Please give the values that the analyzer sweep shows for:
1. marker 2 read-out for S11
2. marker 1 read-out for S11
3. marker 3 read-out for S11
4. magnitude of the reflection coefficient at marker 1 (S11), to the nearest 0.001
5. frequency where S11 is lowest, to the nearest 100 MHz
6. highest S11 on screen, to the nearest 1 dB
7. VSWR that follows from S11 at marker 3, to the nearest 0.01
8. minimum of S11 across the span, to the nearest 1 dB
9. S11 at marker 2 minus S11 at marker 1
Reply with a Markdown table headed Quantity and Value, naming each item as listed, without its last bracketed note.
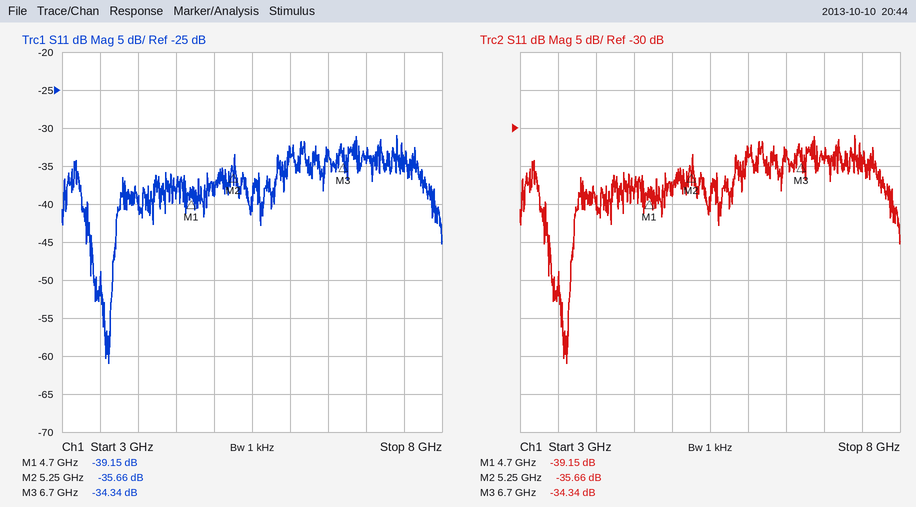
| Quantity | Value |
|---|---|
| marker 2 read-out for S11 | -35.66 dB |
| marker 1 read-out for S11 | -39.15 dB |
| marker 3 read-out for S11 | -34.34 dB |
| magnitude of the reflection coefficient at marker 1 (S11), to the nearest 0.001 | 0.011 |
| frequency where S11 is lowest, to the nearest 100 MHz | 3.6 GHz |
| highest S11 on screen, to the nearest 1 dB | -31 dB |
| VSWR that follows from S11 at marker 3, to the nearest 0.01 | 1.04 |
| minimum of S11 across the span, to the nearest 1 dB | -61 dB |
| S11 at marker 2 minus S11 at marker 1 | 3.49 dB |
